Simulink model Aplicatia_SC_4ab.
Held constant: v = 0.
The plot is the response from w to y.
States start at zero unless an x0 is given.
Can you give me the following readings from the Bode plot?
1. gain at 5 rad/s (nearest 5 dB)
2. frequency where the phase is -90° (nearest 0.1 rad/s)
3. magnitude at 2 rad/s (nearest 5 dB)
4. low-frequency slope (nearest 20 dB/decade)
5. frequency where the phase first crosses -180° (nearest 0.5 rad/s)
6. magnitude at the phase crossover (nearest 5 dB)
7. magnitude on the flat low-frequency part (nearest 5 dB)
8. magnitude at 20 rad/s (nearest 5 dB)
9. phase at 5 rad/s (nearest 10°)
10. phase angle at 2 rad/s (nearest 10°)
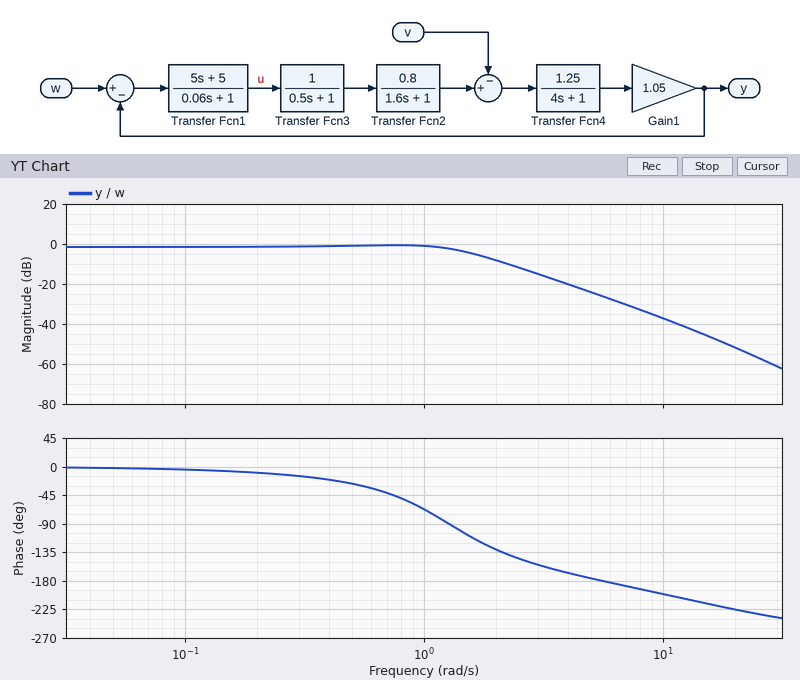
-25 dB
1.3 rad/s
-10 dB
0 dB/decade
5.5 rad/s
-25 dB
0 dB
-50 dB
-180°
-130°
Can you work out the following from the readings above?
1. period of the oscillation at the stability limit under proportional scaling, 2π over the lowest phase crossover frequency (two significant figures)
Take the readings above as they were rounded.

1.1 s
